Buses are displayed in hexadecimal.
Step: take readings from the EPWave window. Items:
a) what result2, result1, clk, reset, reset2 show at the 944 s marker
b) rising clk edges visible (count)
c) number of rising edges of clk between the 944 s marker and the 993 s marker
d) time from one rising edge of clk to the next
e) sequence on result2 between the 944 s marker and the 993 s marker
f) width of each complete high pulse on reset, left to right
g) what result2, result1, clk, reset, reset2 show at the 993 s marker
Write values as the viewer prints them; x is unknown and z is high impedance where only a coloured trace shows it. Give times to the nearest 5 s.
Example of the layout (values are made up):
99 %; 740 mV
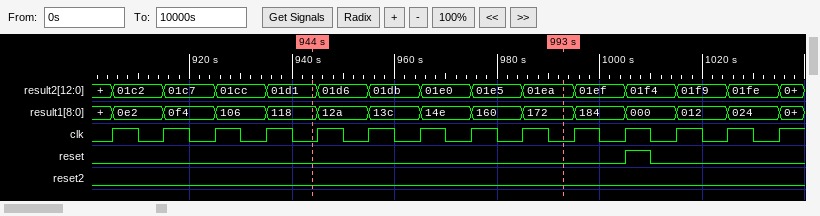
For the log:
result2=01d1, result1=118, clk=0, reset=0, reset2=0; 14; 5; 10 s; 01d1, 01d6, 01db, 01e0, 01e5, 01ea; 5 s; result2=01ea, result1=172, clk=0, reset=0, reset2=0
